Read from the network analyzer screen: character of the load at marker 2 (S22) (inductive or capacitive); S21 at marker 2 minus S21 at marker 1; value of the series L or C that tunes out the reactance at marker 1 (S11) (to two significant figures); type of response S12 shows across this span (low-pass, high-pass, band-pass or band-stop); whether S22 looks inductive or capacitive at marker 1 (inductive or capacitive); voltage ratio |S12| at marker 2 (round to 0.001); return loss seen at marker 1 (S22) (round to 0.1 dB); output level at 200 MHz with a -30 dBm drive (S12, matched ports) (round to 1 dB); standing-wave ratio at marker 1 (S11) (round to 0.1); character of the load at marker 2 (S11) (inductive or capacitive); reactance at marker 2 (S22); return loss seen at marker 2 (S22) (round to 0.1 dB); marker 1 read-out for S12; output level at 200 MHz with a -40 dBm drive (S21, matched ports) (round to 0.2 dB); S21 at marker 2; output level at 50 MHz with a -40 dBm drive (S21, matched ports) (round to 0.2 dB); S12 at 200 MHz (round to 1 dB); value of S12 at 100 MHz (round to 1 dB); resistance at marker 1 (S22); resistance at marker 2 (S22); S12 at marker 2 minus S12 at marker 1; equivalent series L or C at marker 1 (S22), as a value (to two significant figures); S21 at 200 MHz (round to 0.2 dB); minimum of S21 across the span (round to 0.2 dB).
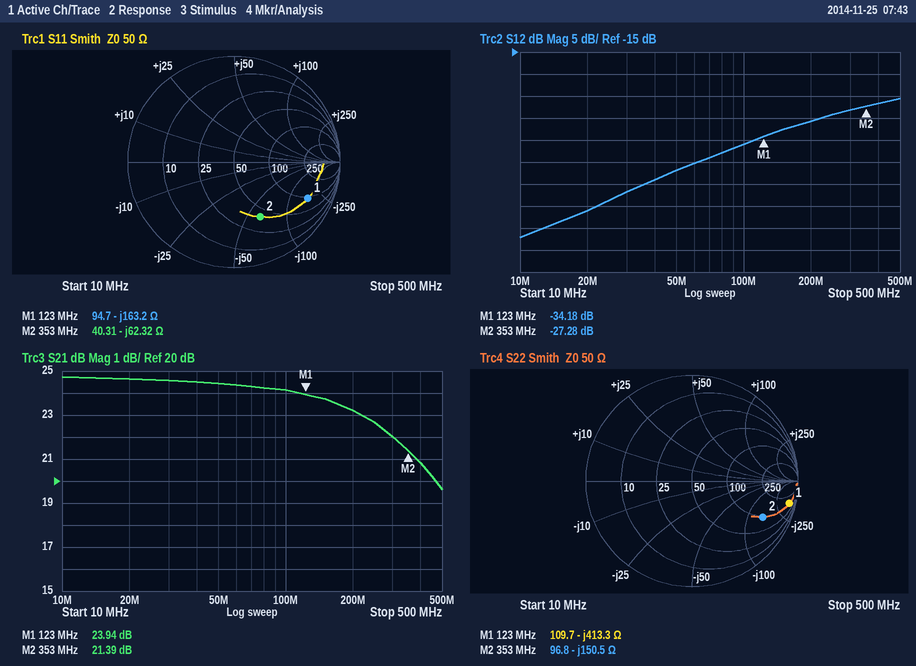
capacitive
-2.55 dB
210 nH
high-pass
capacitive
0.043
0.5 dB
-61 dBm
7.9
capacitive
-150.5 Ω
2.5 dB
-34.18 dB
-16.8 dBm
21.39 dB
-15.6 dBm
-31 dB
-36 dB
109.7 Ω
96.8 Ω
6.90 dB
3.1 pF
23.2 dB
19.6 dB
